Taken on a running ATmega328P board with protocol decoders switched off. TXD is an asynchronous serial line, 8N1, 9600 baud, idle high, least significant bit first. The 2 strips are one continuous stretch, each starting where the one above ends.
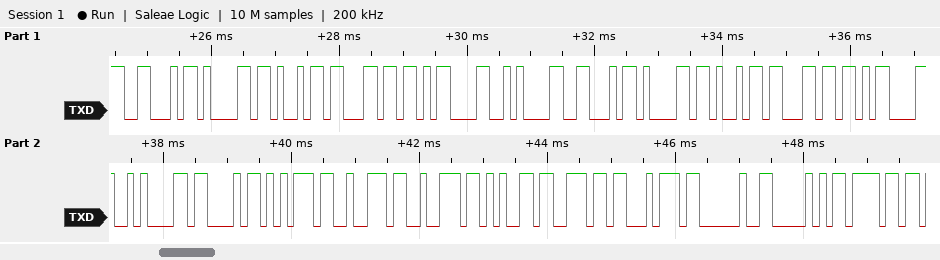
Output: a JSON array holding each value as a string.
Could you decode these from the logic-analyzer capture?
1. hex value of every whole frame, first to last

["0x46 0x61 0x69 0x6C 0x0D 0x0A 0x46 0x61 0x69 0x6C 0x0D 0x0A 0x43 0x75 0x72 0x72 0x65 0x6E 0x74 0x20 0x50 0x6F"]
